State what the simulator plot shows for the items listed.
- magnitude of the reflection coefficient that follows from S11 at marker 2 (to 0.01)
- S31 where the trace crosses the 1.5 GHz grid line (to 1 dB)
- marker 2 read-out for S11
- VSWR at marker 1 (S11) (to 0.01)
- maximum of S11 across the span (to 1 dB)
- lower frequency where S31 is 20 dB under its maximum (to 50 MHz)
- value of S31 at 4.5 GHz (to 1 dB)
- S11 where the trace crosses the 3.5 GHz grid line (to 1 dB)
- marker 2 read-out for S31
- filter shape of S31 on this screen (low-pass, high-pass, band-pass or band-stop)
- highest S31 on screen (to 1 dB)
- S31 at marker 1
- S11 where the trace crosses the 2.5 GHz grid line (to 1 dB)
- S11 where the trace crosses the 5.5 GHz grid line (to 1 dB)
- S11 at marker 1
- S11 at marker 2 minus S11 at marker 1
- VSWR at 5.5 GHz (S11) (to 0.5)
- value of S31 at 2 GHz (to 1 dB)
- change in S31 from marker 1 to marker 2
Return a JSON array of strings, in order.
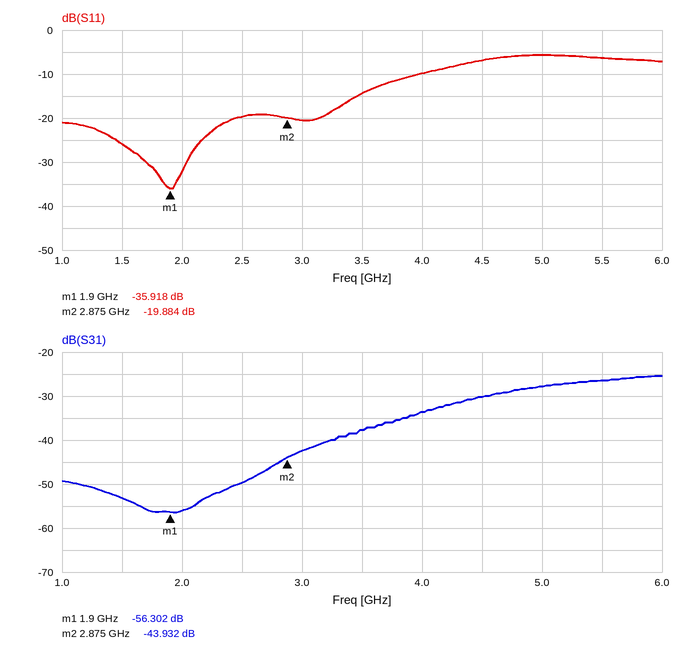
["0.10", "-53 dB", "-19.884 dB", "1.03", "-6 dB", "2.80 GHz", "-30 dB", "-14 dB", "-43.932 dB", "high-pass", "-25 dB", "-56.302 dB", "-20 dB", "-6 dB", "-35.918 dB", "16.034 dB", "3.0", "-56 dB", "12.370 dB"]
